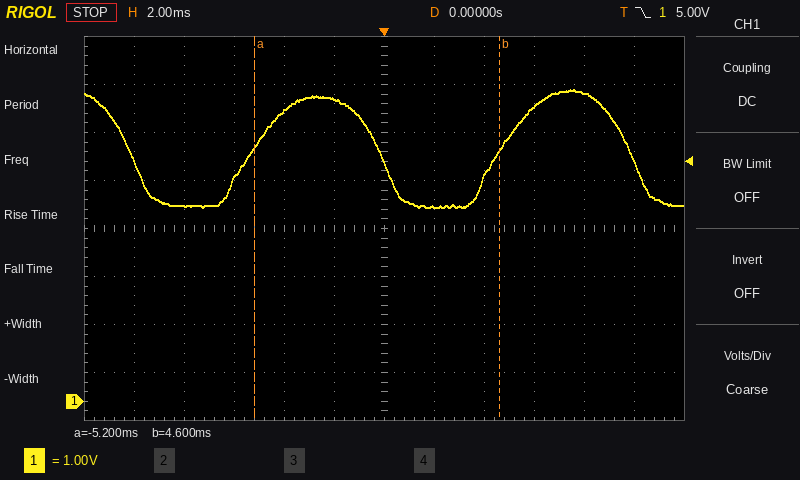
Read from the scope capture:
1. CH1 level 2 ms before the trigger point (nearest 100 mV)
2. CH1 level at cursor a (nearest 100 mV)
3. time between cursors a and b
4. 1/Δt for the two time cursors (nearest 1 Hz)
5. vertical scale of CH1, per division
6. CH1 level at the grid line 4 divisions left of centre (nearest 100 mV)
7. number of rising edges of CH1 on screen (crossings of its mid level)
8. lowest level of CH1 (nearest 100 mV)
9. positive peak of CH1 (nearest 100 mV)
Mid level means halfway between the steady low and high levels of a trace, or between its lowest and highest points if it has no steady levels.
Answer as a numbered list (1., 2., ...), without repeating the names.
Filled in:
1. 6.3 V
2. 5.3 V
3. 9.8 ms
4. 102 Hz
5. 1 V
6. 4.1 V
7. 2
8. 4.0 V
9. 6.5 V
